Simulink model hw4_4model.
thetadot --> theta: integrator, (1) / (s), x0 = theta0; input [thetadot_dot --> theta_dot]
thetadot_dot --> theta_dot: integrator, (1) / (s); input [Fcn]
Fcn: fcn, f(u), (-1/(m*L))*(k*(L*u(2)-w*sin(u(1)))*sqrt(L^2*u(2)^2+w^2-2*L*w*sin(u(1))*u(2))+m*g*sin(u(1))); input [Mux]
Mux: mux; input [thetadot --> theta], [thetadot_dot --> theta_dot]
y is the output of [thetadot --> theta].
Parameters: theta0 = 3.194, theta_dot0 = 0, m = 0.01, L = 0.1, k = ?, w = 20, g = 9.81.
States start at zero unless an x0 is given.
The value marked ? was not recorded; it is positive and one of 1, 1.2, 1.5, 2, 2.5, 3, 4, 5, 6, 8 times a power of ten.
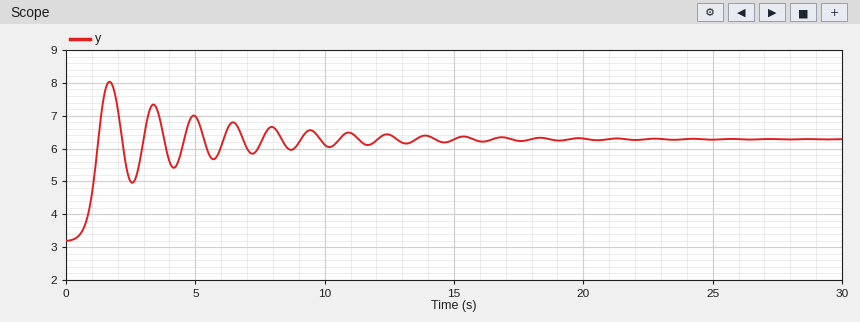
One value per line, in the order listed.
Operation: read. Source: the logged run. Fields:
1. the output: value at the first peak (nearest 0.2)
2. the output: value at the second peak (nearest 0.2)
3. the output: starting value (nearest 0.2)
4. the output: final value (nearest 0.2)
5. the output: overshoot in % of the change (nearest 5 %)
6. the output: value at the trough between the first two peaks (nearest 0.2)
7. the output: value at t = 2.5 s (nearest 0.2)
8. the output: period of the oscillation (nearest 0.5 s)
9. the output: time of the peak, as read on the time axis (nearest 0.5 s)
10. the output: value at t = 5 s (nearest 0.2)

8.0
7.4
3.2
6.2
55 %
5.0
5.0
1.5 s
1.5 s
7.0
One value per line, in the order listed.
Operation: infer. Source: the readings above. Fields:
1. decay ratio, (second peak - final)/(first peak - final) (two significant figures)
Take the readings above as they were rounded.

0.67
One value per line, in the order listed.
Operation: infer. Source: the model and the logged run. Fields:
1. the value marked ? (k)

0.0002
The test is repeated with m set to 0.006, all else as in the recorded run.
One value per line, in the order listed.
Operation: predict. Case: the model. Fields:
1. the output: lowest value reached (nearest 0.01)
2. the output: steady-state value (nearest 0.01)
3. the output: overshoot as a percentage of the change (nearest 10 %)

3.10
3.14
80 %
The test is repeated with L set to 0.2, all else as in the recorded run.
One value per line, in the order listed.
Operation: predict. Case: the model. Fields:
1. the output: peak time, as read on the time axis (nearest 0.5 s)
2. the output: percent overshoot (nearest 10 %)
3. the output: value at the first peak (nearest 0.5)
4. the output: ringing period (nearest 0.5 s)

2.5 s
50 %
8.0
2.5 s
